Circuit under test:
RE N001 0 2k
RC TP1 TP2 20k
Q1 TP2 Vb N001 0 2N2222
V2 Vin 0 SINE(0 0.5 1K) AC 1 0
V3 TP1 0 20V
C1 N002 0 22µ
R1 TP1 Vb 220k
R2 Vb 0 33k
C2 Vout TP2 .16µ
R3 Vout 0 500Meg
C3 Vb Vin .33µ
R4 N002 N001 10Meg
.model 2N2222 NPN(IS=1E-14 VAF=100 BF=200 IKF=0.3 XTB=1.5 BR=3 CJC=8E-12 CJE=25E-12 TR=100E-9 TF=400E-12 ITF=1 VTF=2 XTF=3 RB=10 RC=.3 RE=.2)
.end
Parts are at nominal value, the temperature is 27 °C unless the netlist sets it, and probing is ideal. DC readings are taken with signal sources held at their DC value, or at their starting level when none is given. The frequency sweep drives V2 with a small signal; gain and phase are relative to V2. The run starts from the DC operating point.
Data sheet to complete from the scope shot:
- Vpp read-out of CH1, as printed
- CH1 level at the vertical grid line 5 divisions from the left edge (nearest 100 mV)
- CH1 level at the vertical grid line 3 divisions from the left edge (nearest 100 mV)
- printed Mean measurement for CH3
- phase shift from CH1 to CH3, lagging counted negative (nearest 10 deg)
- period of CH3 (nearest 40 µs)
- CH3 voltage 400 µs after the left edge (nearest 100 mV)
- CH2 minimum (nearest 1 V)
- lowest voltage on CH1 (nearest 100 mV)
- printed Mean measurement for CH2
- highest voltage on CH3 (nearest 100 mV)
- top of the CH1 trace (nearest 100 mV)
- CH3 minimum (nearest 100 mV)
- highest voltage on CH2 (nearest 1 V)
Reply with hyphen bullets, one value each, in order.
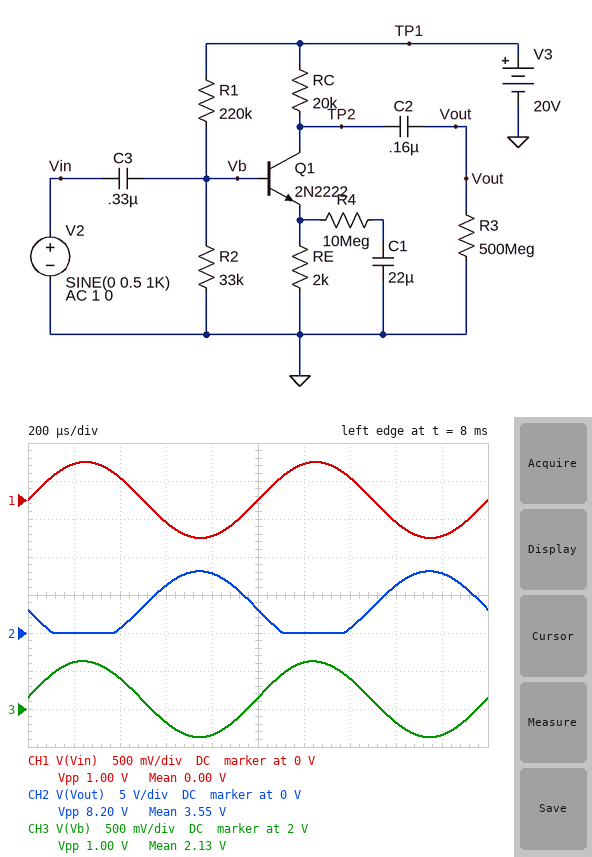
- 1.00 V
- 0 V
- -300 mV
- 2.13 V
- 0 deg
- 1.00 ms
- 2.4 V
- 0 V
- -500 mV
- 3.55 V
- 2.6 V
- 500 mV
- 1.6 V
- 8 V
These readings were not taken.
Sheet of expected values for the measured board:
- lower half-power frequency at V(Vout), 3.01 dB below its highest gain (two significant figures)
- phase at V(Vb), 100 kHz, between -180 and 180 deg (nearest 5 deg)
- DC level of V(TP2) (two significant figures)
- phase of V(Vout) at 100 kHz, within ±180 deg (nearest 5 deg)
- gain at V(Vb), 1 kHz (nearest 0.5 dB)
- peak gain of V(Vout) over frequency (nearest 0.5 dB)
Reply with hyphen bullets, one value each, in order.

- 86 Hz
- 0 deg
- 2.0 V
- 170 deg
- 0 dB
- 16.5 dB
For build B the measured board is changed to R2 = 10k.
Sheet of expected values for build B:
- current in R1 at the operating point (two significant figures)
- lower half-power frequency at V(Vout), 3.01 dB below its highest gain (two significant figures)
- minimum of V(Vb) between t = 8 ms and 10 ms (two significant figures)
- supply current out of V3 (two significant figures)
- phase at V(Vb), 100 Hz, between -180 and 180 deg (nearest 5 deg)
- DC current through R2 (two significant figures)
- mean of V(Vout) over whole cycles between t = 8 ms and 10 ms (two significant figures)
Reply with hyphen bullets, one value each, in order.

- 87 µA
- 51 Hz
- 360 mV
- 220 µA
- 25 deg
- 86 µA
- -430 mV
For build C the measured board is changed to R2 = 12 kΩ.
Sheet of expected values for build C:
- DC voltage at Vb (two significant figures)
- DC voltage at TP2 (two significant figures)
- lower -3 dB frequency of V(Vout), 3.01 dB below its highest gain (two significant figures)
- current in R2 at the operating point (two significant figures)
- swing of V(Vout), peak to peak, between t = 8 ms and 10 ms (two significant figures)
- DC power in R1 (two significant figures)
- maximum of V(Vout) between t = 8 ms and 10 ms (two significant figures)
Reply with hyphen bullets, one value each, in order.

- 1.0 V
- 16 V
- 43 Hz
- 85 µA
- 8.8 V
- 1.6 mW
- 4.0 V
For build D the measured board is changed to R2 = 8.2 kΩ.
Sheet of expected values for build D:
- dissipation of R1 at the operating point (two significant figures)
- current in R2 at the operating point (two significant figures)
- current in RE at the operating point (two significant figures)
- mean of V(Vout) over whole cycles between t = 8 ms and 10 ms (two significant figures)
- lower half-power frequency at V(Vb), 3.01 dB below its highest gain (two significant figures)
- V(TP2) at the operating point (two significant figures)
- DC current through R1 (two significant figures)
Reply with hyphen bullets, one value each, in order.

- 1.7 mW
- 87 µA
- 68 µA
- -830 mV
- 62 Hz
- 19 V
- 88 µA
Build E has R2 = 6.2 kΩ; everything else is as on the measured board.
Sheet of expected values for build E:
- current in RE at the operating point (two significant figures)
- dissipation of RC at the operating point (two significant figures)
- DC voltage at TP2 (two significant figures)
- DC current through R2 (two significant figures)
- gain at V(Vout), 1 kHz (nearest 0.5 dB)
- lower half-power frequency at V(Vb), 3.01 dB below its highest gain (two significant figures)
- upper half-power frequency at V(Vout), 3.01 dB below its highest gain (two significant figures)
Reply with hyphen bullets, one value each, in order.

- 9.3 µA
- 1.7 µW
- 20 V
- 88 µA
- 12.5 dB
- 80 Hz
- 2.7 MHz
